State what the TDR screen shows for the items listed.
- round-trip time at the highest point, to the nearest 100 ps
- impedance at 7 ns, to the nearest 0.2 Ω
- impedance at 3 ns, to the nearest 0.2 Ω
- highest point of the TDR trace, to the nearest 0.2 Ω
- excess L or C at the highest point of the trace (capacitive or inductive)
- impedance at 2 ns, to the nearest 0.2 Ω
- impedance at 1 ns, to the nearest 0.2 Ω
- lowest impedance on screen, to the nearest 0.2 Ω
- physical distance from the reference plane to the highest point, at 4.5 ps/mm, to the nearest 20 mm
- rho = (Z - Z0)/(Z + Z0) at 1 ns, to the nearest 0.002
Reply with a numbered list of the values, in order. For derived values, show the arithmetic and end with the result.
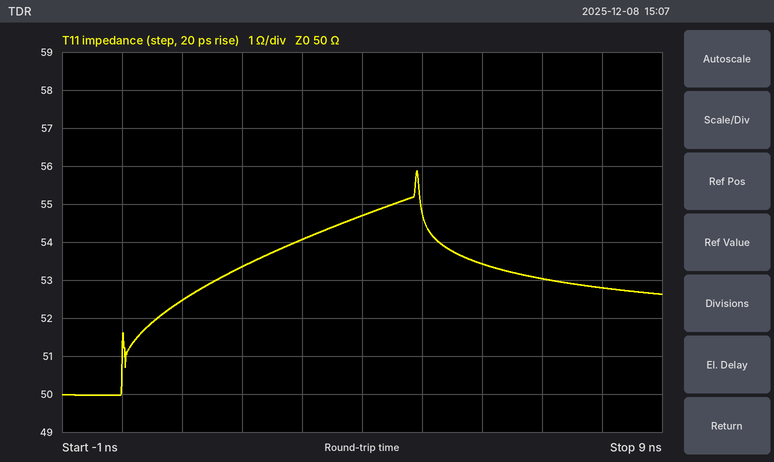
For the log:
1. 4.9 ns
2. 53.0 Ω
3. 54.0 Ω
4. 55.8 Ω
5. inductive
6. 53.4 Ω
7. 52.4 Ω
8. 50.0 Ω
9. 4.9 ns / 2 / 4.5 ps/mm ≈ 544 mm, so 540 mm to the nearest 20 mm
10. (52.4 − 50)/(52.4 + 50) ≈ +0.0234, so +0.024 to the nearest 0.002
